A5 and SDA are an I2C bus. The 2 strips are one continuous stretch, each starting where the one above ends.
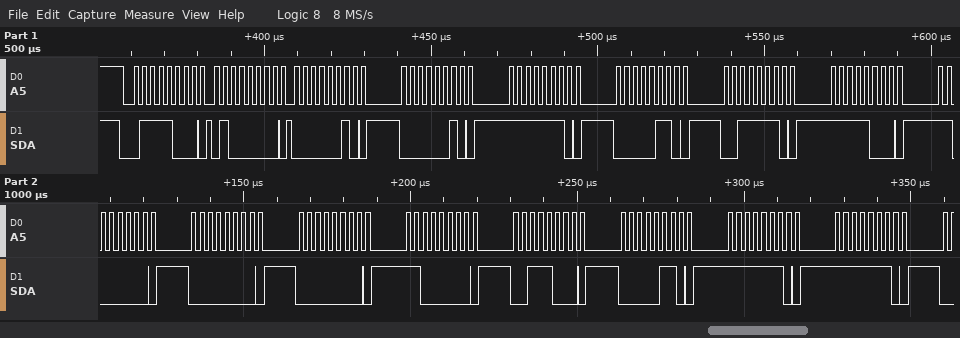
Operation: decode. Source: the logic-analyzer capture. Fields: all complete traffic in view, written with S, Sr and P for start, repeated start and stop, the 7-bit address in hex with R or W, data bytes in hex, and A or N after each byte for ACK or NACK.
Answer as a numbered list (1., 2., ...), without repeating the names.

1. S 3CW A 40 A 02 A 02 A FE A 06 A 3E A F8 A C0 A 00 A 00 A C0 A 38 A 06 A FE A FE A
